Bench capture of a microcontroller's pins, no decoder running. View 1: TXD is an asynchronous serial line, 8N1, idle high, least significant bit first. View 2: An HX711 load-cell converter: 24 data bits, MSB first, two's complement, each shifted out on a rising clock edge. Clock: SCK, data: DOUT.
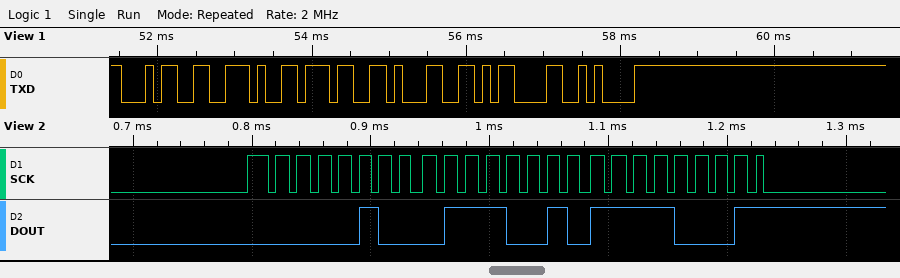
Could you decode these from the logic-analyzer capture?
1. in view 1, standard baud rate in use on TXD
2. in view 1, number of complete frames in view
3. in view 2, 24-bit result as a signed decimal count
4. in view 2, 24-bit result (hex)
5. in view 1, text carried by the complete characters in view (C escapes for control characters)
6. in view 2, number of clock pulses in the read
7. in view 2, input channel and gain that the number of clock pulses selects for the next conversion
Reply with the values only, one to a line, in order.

9600 baud
6
291569
0x0472F1
"4.71\r\n"
25
channel A, gain 128
